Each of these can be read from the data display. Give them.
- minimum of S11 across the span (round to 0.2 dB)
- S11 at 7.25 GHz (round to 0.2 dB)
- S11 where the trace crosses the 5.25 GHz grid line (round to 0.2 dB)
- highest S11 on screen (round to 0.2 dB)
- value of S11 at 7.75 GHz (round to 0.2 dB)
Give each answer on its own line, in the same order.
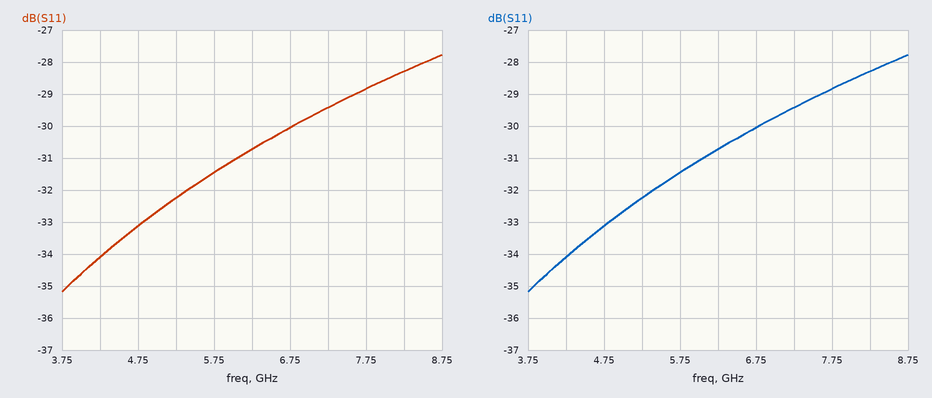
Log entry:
-35.2 dB
-29.4 dB
-32.2 dB
-27.8 dB
-28.8 dB
